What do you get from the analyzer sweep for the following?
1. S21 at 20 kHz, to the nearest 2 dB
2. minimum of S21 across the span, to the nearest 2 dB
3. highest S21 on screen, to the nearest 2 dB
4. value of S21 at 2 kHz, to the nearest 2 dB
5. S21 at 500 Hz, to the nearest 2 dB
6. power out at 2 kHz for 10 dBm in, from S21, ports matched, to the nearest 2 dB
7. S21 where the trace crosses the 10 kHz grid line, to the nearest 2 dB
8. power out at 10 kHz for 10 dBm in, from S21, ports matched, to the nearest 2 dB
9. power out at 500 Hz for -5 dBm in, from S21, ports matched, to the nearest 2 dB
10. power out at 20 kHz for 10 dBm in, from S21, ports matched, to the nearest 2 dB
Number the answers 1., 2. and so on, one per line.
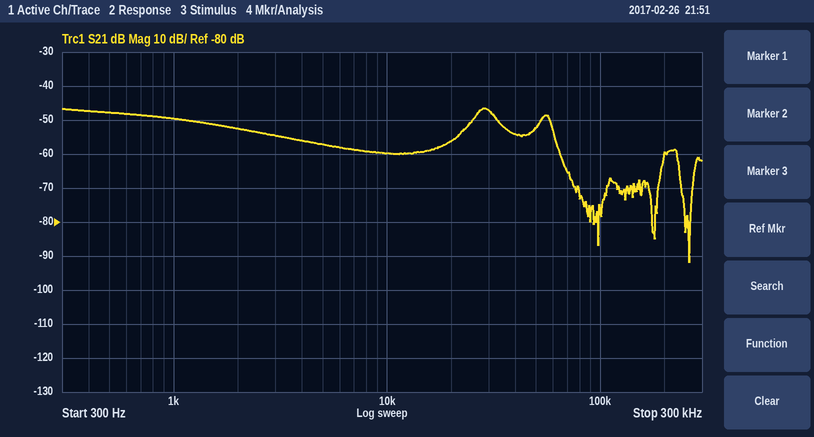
1. -56 dB
2. -92 dB
3. -46 dB
4. -52 dB
5. -48 dB
6. -42 dBm
7. -60 dB
8. -50 dBm
9. -52 dBm
10. -46 dBm
